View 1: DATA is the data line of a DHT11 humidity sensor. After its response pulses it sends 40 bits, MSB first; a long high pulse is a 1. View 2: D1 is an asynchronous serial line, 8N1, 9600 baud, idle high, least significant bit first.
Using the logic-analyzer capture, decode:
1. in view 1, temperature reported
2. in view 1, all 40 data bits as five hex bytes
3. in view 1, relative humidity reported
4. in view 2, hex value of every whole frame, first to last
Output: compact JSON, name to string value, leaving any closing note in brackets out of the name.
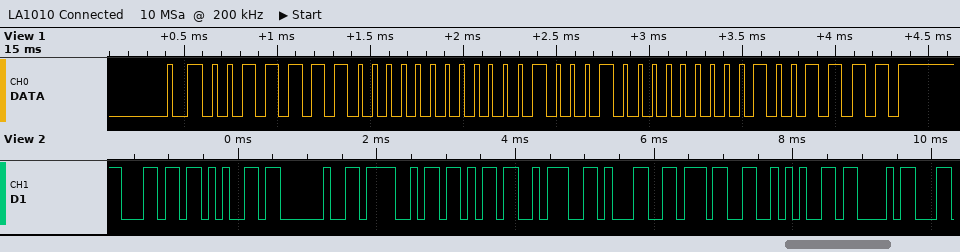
{"in view 1, temperature reported": "17.0 °C", "in view 1, all 40 data bits as five hex bytes": "3E 00 11 00 4F", "in view 1, relative humidity reported": "62 %", "in view 2, hex value of every whole frame, first to last": "0x6C 0x65 0x20 0x4F 0x6B 0x3A 0x31 0x37 0x2A 0x43"}
